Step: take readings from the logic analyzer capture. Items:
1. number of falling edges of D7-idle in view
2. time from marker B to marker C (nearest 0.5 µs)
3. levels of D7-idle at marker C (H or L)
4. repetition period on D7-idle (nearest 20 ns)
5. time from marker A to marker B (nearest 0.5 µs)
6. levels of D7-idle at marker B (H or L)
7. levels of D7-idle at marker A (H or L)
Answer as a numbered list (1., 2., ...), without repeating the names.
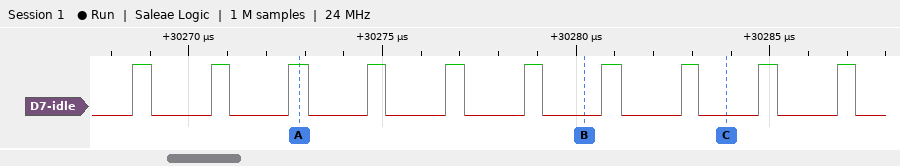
1. 10
2. 3.5 µs
3. D7-idle=L
4. 2020 ns
5. 7.5 µs
6. D7-idle=L
7. D7-idle=H
